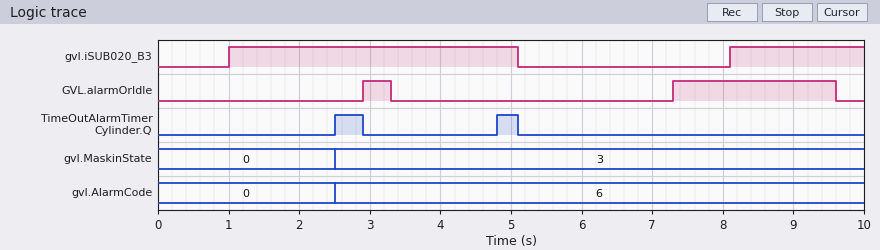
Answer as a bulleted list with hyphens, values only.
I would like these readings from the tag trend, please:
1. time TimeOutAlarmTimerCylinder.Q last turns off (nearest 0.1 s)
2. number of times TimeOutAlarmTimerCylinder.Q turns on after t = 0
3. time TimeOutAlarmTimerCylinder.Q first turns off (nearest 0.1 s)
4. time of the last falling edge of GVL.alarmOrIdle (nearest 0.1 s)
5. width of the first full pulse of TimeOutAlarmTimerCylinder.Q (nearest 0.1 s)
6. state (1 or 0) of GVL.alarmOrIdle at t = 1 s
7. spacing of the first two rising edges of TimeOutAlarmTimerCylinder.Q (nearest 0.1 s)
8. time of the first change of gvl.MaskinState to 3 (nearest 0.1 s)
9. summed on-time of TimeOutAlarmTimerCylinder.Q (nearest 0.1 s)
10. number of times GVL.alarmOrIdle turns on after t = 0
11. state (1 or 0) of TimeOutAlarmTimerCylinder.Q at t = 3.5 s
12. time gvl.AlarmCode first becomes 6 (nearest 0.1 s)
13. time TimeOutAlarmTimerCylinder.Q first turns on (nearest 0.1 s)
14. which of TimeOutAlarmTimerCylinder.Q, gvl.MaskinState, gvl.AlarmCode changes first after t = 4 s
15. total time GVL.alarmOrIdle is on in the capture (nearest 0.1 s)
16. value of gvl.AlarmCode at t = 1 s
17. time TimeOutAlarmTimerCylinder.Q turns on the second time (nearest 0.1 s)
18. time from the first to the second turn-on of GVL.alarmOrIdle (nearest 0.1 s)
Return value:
- 5.1 s
- 2
- 2.9 s
- 9.6 s
- 0.4 s
- 0
- 2.3 s
- 2.5 s
- 0.7 s
- 2
- 0
- 2.5 s
- 2.5 s
- TimeOutAlarmTimerCylinder.Q
- 2.7 s
- 0
- 4.8 s
- 4.4 s
